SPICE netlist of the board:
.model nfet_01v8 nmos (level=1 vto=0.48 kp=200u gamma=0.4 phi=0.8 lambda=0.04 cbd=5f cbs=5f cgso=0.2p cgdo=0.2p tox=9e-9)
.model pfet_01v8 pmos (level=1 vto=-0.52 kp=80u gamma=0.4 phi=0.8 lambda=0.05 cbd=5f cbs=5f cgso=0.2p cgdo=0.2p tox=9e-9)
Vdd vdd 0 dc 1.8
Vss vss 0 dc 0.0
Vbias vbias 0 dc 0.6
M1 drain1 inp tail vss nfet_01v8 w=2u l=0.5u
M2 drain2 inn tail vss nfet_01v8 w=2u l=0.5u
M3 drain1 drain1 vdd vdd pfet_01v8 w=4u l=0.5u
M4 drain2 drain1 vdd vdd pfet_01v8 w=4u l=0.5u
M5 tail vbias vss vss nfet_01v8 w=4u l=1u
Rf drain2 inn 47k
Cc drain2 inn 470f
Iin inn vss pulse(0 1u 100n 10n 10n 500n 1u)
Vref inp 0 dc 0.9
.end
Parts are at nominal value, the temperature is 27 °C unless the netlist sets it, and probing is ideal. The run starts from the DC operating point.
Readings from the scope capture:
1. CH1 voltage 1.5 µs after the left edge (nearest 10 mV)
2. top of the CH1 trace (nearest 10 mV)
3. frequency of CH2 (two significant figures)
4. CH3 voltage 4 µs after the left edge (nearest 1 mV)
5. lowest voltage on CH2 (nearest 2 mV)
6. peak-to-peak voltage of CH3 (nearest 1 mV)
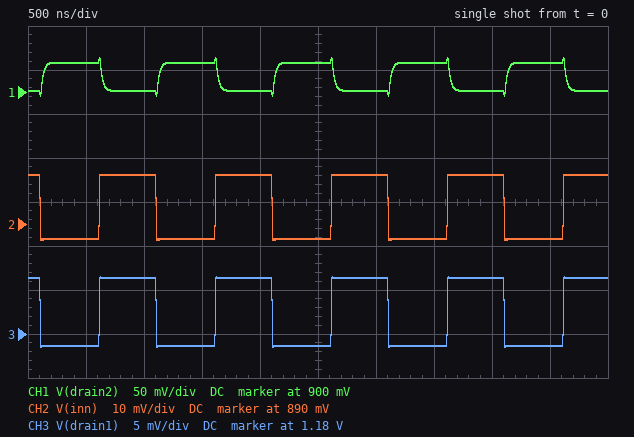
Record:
930 mV
940 mV
1.0 MHz
1.186 V
886 mV
8 mV
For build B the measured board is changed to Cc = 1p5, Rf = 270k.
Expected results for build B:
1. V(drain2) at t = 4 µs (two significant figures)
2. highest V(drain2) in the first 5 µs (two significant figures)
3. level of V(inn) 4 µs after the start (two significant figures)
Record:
980 mV
1.1 V
900 mV
